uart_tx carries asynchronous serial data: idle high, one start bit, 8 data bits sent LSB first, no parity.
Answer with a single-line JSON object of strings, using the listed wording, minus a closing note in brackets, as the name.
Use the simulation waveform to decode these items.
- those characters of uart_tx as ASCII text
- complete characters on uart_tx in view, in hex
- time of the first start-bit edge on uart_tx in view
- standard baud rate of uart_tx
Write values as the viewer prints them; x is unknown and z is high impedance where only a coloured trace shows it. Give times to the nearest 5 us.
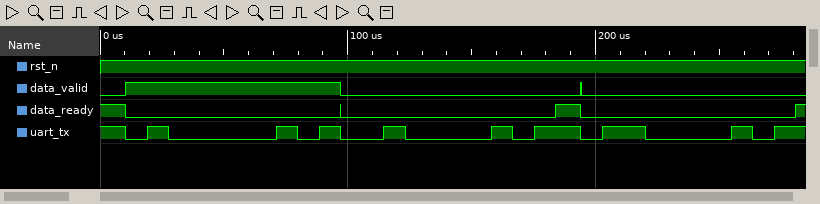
{"those characters of uart_tx as ASCII text": "\"ABC\"", "complete characters on uart_tx in view, in hex": "41, 42, 43", "time of the first start-bit edge on uart_tx in view": "10 us", "standard baud rate of uart_tx": "115200 baud"}
